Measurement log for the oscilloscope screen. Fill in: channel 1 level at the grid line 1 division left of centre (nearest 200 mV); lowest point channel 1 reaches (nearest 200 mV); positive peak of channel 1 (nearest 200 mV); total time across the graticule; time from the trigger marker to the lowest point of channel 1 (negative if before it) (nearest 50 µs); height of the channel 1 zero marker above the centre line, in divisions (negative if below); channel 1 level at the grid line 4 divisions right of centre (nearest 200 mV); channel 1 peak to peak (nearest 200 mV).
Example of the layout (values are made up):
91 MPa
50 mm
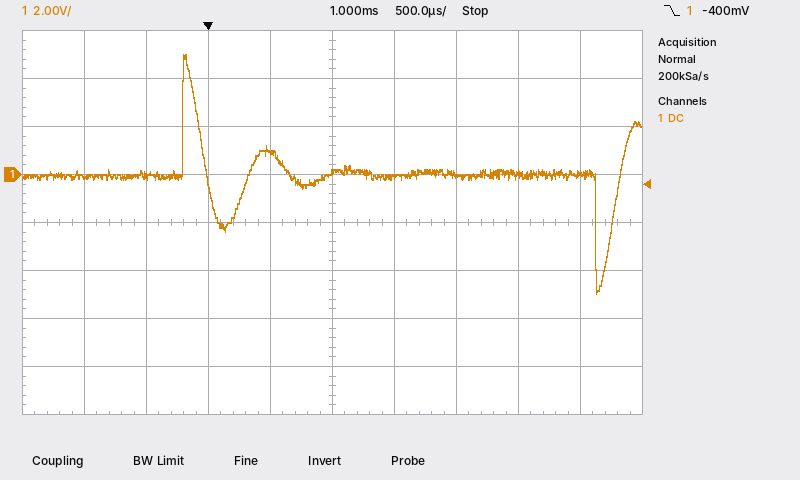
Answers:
1.0 V
-5.0 V
5.0 V
5 ms
+3.15 ms
+1.0 div
0.0 V
10.0 V
